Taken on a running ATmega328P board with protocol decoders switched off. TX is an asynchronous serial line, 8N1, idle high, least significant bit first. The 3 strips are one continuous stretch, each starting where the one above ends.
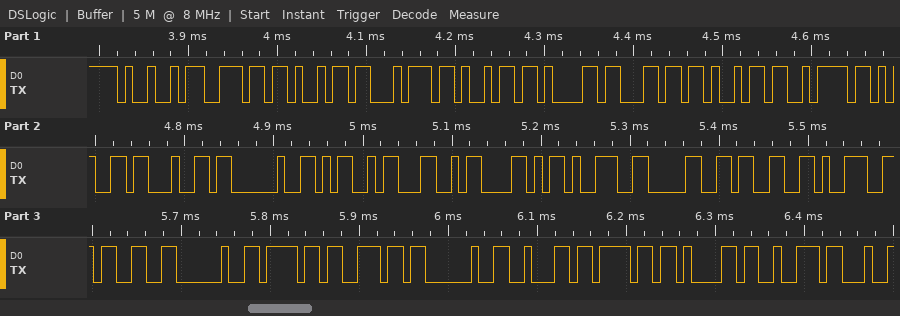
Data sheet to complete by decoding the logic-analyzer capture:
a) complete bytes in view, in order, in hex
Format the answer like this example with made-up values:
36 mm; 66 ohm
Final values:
0x49 0x6E 0x69 0x74 0x69 0x61 0x6C 0x69 0x7A 0x65 0x64 0x20 0x4D 0x4C 0x58 0x39 0x30 0x33 0x39 0x33 0x20 0x6F 0x6E 0x20 0x62 0x6F 0x61 0x72
